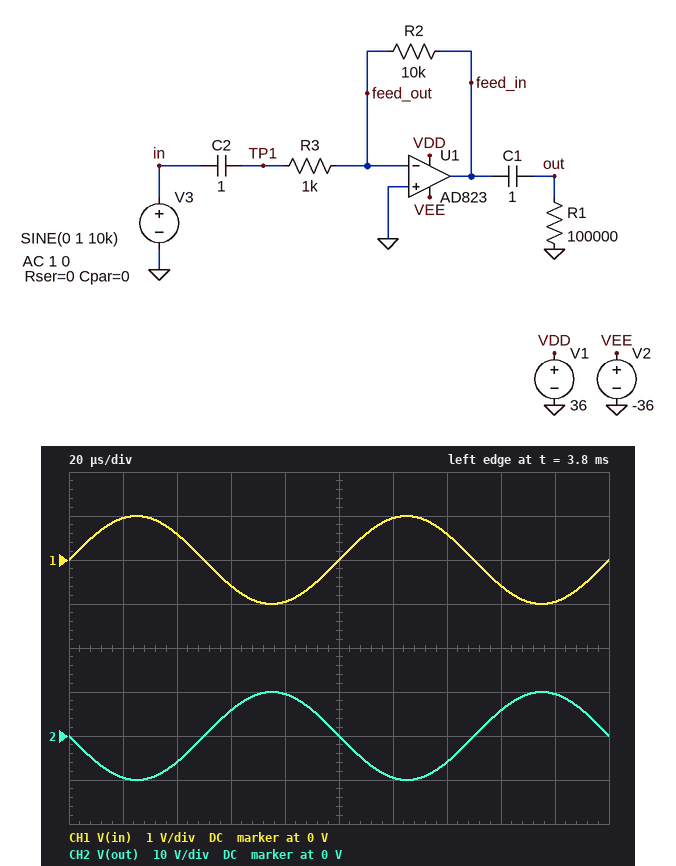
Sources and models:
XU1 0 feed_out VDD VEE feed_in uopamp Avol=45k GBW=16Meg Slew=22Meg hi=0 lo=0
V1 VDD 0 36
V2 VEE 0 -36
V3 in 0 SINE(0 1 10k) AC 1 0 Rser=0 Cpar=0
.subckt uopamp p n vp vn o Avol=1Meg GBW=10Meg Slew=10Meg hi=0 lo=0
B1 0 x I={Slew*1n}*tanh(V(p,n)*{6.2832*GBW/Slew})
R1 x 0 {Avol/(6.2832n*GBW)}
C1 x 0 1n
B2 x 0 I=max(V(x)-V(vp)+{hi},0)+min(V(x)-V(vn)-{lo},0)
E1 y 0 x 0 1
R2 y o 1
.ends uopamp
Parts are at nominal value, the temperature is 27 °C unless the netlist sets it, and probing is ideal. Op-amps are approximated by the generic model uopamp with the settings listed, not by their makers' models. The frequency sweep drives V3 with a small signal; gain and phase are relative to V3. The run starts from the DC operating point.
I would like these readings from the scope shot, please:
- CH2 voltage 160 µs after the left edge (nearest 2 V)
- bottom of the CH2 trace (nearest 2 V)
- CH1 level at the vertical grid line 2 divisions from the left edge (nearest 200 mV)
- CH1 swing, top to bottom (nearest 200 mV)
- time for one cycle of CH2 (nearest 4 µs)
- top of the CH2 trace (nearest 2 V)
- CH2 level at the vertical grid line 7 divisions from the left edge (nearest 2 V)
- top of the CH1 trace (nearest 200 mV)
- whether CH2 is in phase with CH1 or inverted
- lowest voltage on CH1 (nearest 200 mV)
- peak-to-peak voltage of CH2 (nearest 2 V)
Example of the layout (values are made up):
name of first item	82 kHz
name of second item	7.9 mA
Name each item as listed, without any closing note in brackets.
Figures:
CH2 voltage 160 µs after the left edge	6 V
bottom of the CH2 trace	-10 V
CH1 level at the vertical grid line 2 divisions from the left edge	600 mV
CH1 swing, top to bottom	2.0 V
time for one cycle of CH2	100 µs
top of the CH2 trace	10 V
CH2 level at the vertical grid line 7 divisions from the left edge	-6 V
top of the CH1 trace	1.0 V
whether CH2 is in phase with CH1 or inverted	inverted
lowest voltage on CH1	-1.0 V
peak-to-peak voltage of CH2	20 V
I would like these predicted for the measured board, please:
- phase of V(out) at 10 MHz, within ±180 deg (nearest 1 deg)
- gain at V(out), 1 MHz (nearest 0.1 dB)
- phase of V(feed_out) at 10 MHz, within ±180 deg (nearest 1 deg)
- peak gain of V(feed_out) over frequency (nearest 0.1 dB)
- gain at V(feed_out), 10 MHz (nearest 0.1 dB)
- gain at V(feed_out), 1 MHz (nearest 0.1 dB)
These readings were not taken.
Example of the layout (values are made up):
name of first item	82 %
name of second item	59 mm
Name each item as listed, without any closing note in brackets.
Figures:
phase of V(out) at 10 MHz, within ±180 deg	98 deg
gain at V(out), 1 MHz	18.3 dB
phase of V(feed_out) at 10 MHz, within ±180 deg	8 deg
peak gain of V(feed_out) over frequency	-0.8 dB
gain at V(feed_out), 10 MHz	-0.9 dB
gain at V(feed_out), 1 MHz	-5.8 dB
